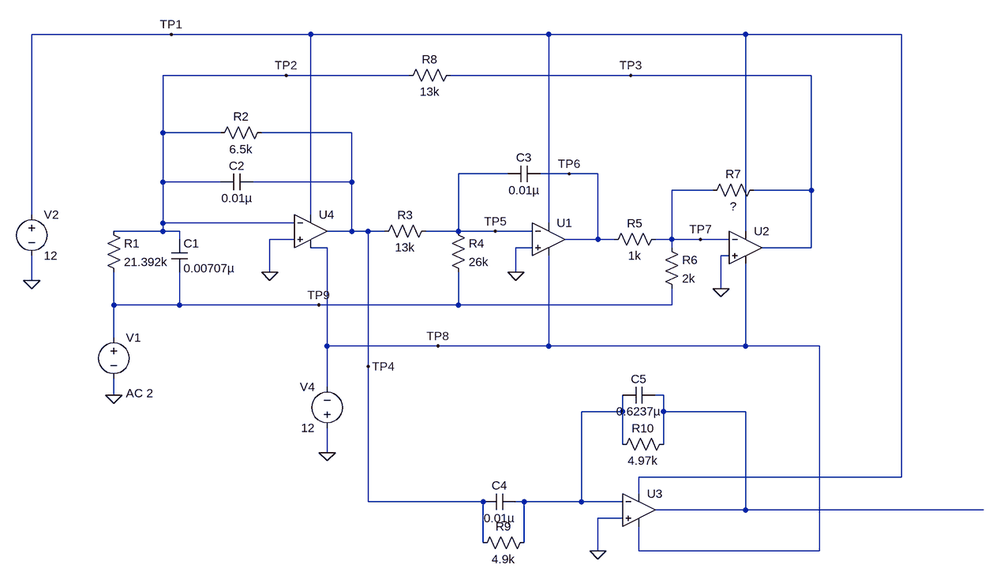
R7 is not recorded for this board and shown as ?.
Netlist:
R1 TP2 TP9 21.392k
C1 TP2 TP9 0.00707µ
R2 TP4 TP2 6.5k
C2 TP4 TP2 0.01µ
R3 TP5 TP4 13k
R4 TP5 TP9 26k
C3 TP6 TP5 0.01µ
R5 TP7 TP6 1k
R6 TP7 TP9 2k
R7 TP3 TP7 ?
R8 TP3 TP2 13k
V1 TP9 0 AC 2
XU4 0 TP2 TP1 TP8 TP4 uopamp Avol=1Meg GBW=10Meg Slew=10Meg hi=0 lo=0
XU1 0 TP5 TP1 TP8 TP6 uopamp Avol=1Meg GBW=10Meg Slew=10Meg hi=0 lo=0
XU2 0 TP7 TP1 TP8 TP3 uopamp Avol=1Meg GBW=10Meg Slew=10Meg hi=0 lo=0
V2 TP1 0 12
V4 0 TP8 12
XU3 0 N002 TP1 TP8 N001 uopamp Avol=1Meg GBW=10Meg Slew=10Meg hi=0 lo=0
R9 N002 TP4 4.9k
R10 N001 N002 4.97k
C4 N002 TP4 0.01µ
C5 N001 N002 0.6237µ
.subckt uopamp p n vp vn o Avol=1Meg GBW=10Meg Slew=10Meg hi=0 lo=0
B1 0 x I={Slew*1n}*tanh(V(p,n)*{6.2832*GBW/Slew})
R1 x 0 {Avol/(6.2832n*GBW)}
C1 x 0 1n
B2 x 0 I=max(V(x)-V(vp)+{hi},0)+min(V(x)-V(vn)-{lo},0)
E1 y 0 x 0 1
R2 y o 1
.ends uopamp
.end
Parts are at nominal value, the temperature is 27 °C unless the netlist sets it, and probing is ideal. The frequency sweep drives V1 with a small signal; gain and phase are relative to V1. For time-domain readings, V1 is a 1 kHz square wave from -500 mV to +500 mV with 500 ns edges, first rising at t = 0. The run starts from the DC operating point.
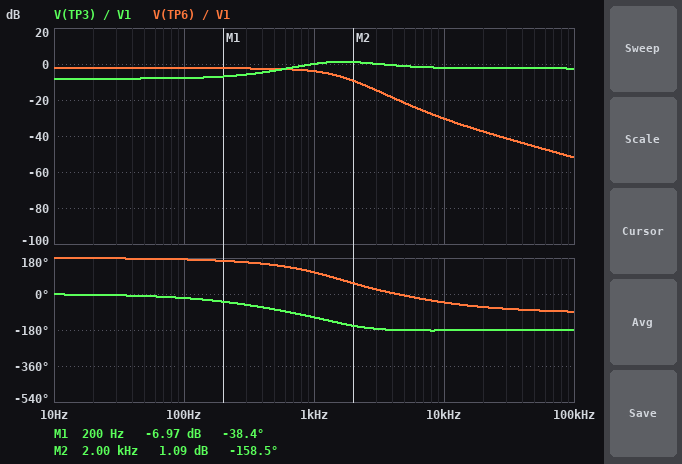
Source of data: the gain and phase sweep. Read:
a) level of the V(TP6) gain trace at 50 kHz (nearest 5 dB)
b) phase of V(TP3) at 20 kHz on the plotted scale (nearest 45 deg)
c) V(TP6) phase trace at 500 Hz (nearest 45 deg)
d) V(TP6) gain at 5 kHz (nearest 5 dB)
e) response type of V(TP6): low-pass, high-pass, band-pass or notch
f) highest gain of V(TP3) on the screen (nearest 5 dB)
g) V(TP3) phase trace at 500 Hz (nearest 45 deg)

-45 dB
-180 deg
135 deg
-20 dB
low-pass
0 dB
-90 deg
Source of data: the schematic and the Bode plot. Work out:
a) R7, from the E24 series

1.5 kΩ
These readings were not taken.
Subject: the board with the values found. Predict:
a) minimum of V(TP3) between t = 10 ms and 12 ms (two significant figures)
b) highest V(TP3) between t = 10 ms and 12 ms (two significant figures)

-980 mV
980 mV
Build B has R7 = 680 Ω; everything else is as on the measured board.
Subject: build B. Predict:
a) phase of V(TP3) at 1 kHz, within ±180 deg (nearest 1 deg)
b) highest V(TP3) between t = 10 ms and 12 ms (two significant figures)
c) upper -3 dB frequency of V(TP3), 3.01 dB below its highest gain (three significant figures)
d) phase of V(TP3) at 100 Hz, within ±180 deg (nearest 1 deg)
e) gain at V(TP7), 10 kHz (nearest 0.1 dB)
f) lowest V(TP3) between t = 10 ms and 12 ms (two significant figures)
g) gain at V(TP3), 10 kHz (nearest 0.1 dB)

-143 deg
390 mV
7.27 kHz
-28 deg
-69.1 dB
-390 mV
-9.1 dB
